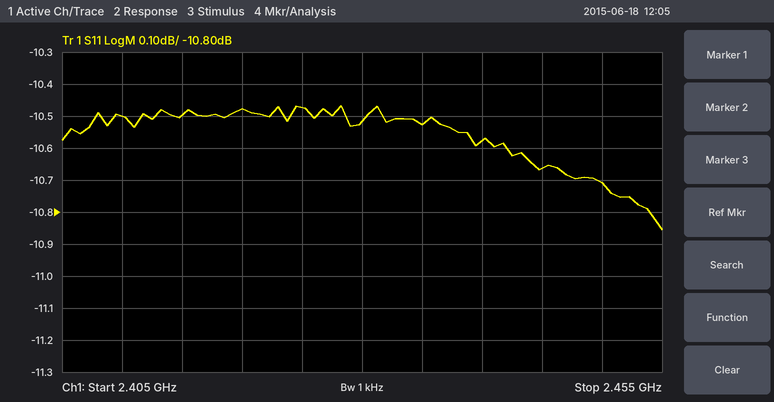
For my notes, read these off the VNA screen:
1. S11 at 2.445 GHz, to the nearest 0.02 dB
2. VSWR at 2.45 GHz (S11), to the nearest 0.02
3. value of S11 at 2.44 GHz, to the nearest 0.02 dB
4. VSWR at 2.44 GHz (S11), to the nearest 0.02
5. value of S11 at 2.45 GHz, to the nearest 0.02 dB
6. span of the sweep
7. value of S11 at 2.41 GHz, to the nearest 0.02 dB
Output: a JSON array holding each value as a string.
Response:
["-10.66 dB", "1.82", "-10.58 dB", "1.84", "-10.70 dB", "50 MHz", "-10.50 dB"]
